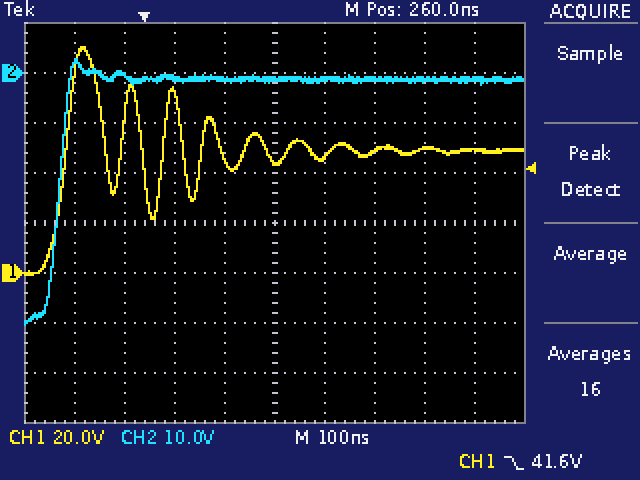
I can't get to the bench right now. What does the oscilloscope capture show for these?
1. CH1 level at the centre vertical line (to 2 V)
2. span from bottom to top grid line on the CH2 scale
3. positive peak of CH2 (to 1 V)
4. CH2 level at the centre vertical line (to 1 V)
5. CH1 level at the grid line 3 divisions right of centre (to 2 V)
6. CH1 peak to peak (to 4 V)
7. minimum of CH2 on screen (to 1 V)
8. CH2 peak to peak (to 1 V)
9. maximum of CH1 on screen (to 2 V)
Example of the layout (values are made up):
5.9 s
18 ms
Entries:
44 V
80 V
3 V
-1 V
50 V
92 V
-50 V
53 V
90 V
